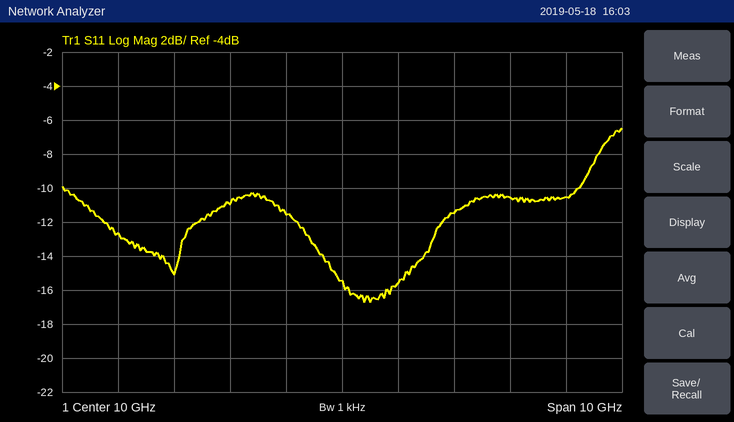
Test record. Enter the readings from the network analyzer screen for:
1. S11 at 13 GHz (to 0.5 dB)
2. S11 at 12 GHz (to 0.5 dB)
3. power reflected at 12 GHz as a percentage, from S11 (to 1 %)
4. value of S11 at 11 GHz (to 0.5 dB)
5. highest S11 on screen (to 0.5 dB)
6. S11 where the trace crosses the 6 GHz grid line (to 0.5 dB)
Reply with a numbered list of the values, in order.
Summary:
1. -10.5 dB
2. -11.5 dB
3. 7 %
4. -15.5 dB
5. -6.5 dB
6. -12.5 dB
